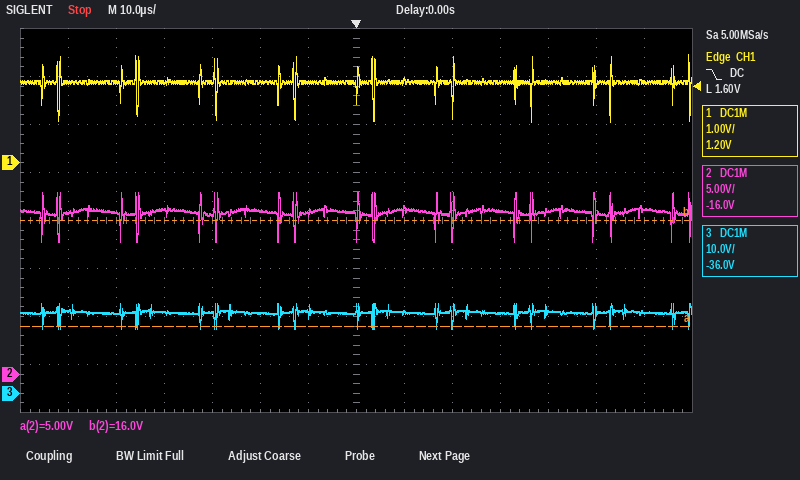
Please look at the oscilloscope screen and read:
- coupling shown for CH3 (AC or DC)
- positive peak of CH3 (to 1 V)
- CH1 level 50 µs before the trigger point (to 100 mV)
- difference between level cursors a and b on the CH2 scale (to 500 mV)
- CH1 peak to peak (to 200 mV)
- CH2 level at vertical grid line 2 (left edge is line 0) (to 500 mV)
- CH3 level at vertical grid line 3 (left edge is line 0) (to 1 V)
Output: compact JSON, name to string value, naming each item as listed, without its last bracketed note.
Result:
{"coupling shown for CH3": "DC", "positive peak of CH3": "19 V", "CH1 level 50 µs before the trigger point": "1.7 V", "difference between level cursors a and b on the CH2 scale": "11.0 V", "CH1 peak to peak": "1.4 V", "CH2 level at vertical grid line 2 (left edge is line 0)": "17.0 V", "CH3 level at vertical grid line 3 (left edge is line 0)": "17 V"}
